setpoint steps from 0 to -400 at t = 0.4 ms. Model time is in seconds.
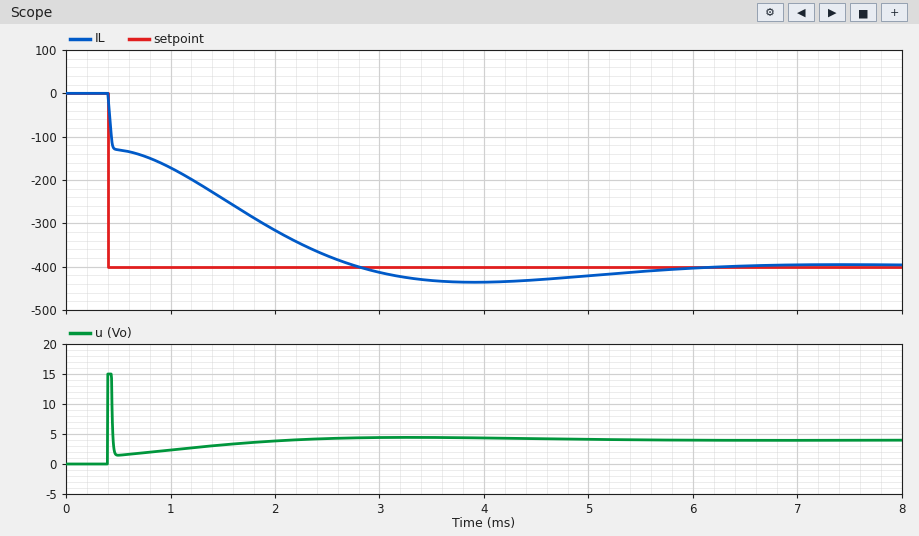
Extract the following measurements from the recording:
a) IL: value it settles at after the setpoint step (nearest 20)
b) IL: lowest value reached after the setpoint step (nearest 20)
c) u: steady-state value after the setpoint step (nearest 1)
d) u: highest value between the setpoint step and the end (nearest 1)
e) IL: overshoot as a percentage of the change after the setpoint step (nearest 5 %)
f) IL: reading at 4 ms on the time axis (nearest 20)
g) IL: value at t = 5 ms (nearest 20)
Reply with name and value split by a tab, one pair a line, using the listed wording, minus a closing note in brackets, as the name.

IL: value it settles at after the setpoint step	-400
IL: lowest value reached after the setpoint step	-440
u: steady-state value after the setpoint step	4
u: highest value between the setpoint step and the end	15
IL: overshoot as a percentage of the change after the setpoint step	10 %
IL: reading at 4 ms on the time axis	-440
IL: value at t = 5 ms	-420
